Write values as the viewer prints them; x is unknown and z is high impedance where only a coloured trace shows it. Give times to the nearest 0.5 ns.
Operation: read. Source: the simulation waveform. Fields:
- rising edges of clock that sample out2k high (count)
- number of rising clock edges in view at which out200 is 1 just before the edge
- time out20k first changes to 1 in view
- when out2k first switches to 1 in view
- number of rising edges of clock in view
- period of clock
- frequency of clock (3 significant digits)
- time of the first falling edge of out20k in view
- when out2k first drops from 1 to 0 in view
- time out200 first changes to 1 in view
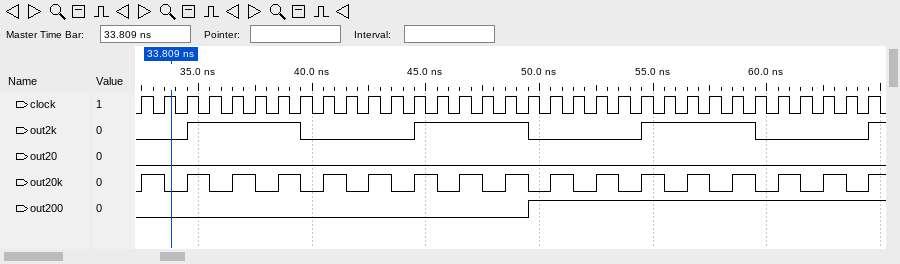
15
15
32.5 ns
34.5 ns
33
1 ns
1.00 GHz
33.5 ns
39.5 ns
49.5 ns
